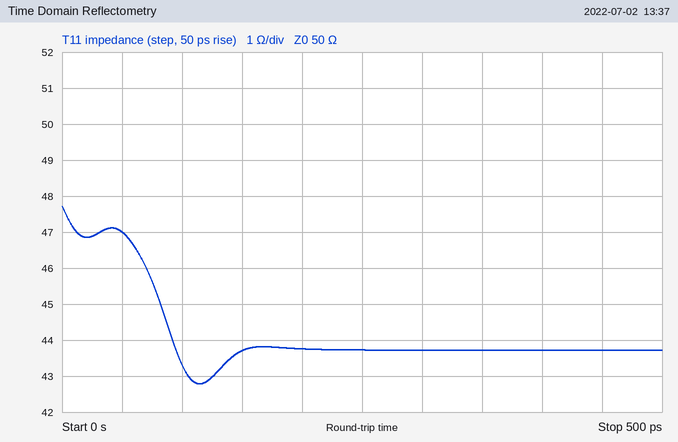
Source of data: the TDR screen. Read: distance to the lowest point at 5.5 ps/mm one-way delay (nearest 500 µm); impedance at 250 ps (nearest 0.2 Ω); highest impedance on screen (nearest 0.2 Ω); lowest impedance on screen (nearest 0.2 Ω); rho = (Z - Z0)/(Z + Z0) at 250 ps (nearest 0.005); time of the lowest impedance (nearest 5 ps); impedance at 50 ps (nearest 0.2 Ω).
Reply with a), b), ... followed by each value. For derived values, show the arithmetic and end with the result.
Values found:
a) 115 ps / 2 / 5.5 ps/mm ≈ 10.5 mm
b) 43.8 Ω
c) 47.8 Ω
d) 42.8 Ω
e) (43.8 − 50)/(43.8 + 50) ≈ -0.0661, so -0.065 to the nearest 0.005
f) 115 ps
g) 47.0 Ω
